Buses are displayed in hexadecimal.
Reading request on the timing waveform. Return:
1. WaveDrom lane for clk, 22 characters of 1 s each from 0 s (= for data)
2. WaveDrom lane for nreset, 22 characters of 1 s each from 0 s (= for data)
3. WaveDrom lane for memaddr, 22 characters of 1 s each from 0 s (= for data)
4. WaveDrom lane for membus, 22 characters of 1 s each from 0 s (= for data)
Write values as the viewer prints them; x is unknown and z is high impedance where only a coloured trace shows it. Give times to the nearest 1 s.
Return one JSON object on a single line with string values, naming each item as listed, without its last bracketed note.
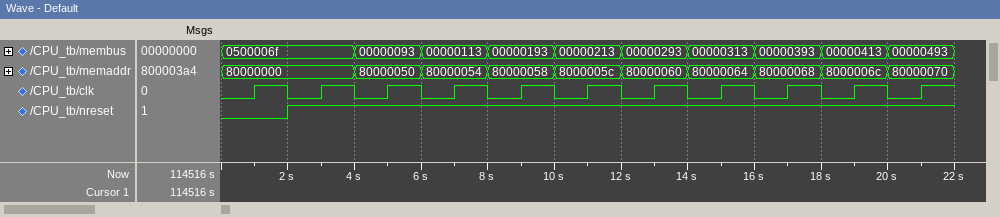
{"WaveDrom lane for clk, 22 characters of 1 s each from 0 s": "{name: 'clk', wave: '0101010101010101010101'}", "WaveDrom lane for nreset, 22 characters of 1 s each from 0 s": "{name: 'nreset', wave: '0.1...................'}", "WaveDrom lane for memaddr, 22 characters of 1 s each from 0 s": "{name: 'memaddr', wave: '=...=.=.=.=.=.=.=.=.=.', data: '80000000 80000050 80000054 80000058 8000005c 80000060 80000064 80000068 8000006c 80000070'}", "WaveDrom lane for membus, 22 characters of 1 s each from 0 s": "{name: 'membus', wave: '=...=.=.=.=.=.=.=.=.=.', data: '0500006f 00000093 00000113 00000193 00000213 00000293 00000313 00000393 00000413 00000493'}"}
